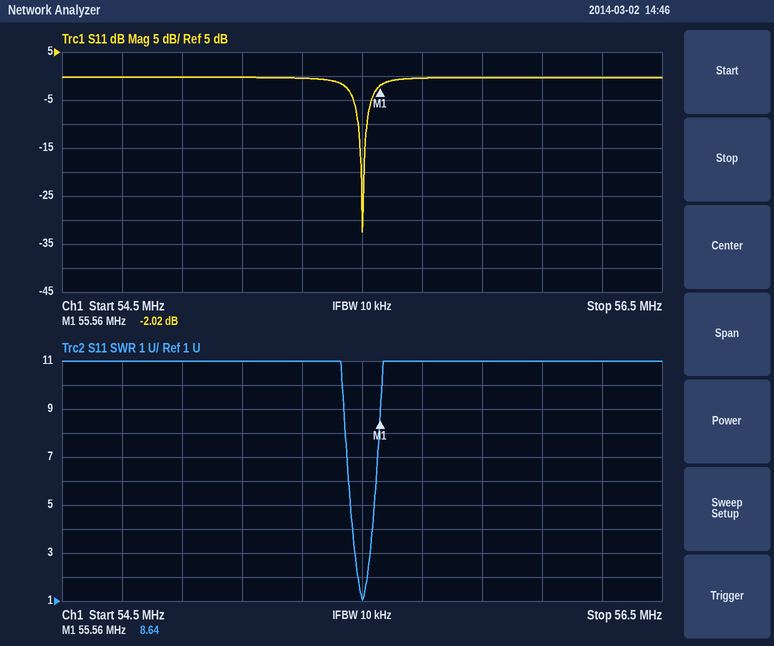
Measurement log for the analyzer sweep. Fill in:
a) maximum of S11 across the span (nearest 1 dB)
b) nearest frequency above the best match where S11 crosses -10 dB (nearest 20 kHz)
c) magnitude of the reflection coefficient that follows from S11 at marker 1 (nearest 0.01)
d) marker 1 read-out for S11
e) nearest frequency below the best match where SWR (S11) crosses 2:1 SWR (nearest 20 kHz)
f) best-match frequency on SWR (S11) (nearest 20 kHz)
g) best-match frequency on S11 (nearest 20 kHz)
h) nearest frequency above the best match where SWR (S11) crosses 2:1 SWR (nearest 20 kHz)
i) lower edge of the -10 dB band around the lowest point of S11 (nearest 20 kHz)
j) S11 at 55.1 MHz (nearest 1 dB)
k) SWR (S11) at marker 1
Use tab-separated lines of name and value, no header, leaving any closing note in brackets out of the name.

maximum of S11 across the span	0 dB
nearest frequency above the best match where S11 crosses -10 dB	55.52 MHz
magnitude of the reflection coefficient that follows from S11 at marker 1	0.79
marker 1 read-out for S11	-2.02 dB
nearest frequency below the best match where SWR (S11) crosses 2:1 SWR	55.48 MHz
best-match frequency on SWR (S11)	55.50 MHz
best-match frequency on S11	55.50 MHz
nearest frequency above the best match where SWR (S11) crosses 2:1 SWR	55.52 MHz
lower edge of the -10 dB band around the lowest point of S11	55.48 MHz
S11 at 55.1 MHz	0 dB
SWR (S11) at marker 1	8.64
